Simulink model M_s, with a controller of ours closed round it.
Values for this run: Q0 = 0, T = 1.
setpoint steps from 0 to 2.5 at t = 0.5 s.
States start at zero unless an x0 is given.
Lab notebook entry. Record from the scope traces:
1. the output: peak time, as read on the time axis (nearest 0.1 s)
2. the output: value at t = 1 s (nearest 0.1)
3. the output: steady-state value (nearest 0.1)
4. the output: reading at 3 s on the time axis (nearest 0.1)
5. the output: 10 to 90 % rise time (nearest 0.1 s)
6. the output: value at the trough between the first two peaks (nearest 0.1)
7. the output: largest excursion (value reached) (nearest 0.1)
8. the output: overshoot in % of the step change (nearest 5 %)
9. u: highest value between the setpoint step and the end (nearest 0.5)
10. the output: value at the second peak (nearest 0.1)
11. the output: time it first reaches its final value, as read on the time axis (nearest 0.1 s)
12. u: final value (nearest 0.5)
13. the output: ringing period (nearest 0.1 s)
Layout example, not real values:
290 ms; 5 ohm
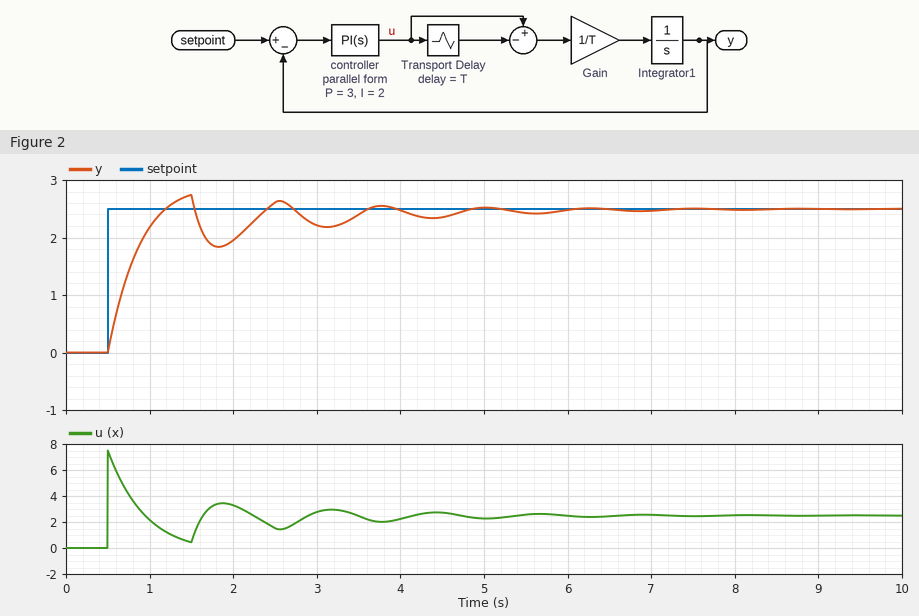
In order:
1.5 s; 2.2; 2.5; 2.2; 0.5 s; 1.8; 2.7; 10 %; 7.5; 2.6; 1.2 s; 2.5; 1.1 s
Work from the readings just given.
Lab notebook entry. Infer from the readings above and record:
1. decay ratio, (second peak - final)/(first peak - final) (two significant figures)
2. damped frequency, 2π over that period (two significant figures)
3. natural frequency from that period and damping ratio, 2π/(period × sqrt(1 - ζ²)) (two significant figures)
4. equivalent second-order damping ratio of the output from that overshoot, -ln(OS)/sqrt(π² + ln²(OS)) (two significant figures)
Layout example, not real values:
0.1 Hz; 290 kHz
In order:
0.50; 5.7 rad/s; 7.1 rad/s; 0.59
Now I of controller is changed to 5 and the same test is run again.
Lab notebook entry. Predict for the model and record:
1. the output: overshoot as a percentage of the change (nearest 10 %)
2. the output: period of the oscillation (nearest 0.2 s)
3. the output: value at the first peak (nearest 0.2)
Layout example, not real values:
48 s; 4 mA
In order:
20 %; 1.0 s; 3.0
